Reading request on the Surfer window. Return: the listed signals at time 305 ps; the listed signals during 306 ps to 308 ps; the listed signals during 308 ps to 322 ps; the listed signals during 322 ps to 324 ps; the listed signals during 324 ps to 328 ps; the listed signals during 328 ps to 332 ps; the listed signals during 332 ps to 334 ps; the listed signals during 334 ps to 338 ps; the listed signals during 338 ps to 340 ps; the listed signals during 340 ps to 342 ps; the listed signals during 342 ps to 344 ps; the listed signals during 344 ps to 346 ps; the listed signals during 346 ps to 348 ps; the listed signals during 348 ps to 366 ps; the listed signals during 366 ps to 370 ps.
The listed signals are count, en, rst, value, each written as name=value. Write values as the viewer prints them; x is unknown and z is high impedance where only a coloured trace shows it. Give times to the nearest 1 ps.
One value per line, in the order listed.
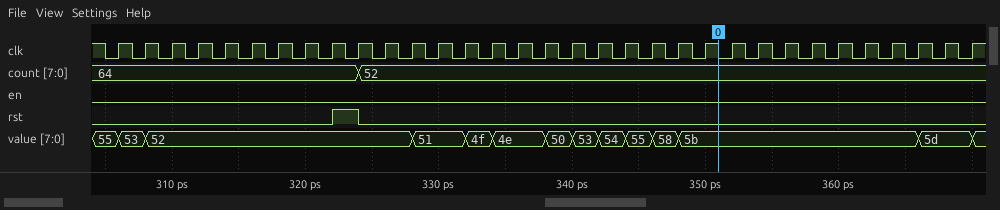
count=64, en=0, rst=0, value=55
count=64, en=0, rst=0, value=53
count=64, en=0, rst=0, value=52
count=64, en=0, rst=1, value=52
count=52, en=0, rst=0, value=52
count=52, en=0, rst=0, value=51
count=52, en=0, rst=0, value=4f
count=52, en=0, rst=0, value=4e
count=52, en=0, rst=0, value=50
count=52, en=0, rst=0, value=53
count=52, en=0, rst=0, value=54
count=52, en=0, rst=0, value=55
count=52, en=0, rst=0, value=58
count=52, en=0, rst=0, value=5b
count=52, en=0, rst=0, value=5d
